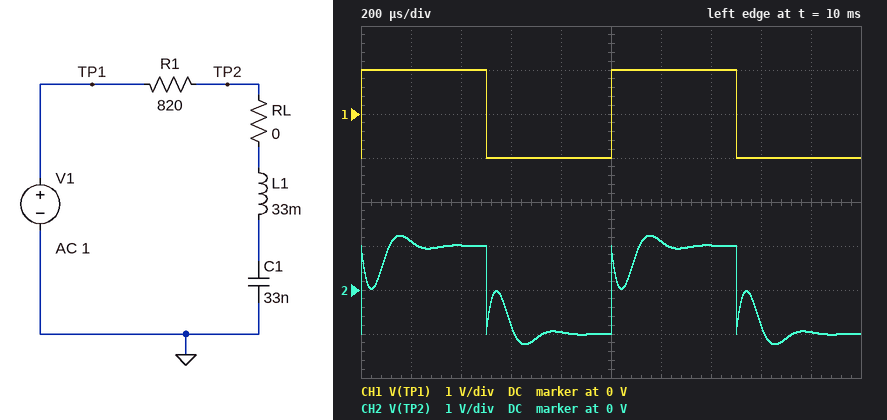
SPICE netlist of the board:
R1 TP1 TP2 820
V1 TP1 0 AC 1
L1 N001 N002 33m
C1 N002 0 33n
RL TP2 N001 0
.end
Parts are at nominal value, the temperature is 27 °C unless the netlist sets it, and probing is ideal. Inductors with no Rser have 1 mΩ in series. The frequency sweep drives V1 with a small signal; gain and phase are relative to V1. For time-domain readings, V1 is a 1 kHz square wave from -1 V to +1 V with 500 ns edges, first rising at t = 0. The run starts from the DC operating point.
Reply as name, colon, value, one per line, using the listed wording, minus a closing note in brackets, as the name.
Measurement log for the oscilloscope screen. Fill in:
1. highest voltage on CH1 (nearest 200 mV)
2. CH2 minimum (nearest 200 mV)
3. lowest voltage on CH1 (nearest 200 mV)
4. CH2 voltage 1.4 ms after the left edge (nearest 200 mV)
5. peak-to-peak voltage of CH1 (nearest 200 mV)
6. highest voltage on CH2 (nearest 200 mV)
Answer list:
highest voltage on CH1: 1.0 V
CH2 minimum: -1.2 V
lowest voltage on CH1: -1.0 V
CH2 voltage 1.4 ms after the left edge: 1.0 V
peak-to-peak voltage of CH1: 2.0 V
highest voltage on CH2: 1.2 V
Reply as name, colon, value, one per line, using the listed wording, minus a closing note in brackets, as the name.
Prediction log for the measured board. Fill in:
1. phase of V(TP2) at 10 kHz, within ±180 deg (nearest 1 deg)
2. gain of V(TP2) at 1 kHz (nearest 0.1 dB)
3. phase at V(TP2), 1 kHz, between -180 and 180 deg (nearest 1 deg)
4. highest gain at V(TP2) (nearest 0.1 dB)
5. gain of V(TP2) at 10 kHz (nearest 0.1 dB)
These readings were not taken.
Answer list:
phase of V(TP2) at 10 kHz, within ±180 deg: 27 deg
gain of V(TP2) at 1 kHz: -0.1 dB
phase at V(TP2), 1 kHz, between -180 and 180 deg: -10 deg
highest gain at V(TP2): 0 dB
gain of V(TP2) at 10 kHz: -1.0 dB
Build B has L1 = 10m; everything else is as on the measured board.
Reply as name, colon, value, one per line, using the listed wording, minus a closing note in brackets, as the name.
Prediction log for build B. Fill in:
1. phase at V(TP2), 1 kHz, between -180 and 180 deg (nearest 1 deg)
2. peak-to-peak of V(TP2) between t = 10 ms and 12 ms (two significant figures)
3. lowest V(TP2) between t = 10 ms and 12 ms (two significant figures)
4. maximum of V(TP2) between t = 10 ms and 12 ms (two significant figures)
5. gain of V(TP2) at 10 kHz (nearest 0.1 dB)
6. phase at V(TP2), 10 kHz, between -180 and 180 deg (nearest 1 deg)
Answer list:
phase at V(TP2), 1 kHz, between -180 and 180 deg: -10 deg
peak-to-peak of V(TP2) between t = 10 ms and 12 ms: 2.1 V
lowest V(TP2) between t = 10 ms and 12 ms: -1.0 V
maximum of V(TP2) between t = 10 ms and 12 ms: 1.0 V
gain of V(TP2) at 10 kHz: -15.1 dB
phase at V(TP2), 10 kHz, between -180 and 180 deg: 80 deg
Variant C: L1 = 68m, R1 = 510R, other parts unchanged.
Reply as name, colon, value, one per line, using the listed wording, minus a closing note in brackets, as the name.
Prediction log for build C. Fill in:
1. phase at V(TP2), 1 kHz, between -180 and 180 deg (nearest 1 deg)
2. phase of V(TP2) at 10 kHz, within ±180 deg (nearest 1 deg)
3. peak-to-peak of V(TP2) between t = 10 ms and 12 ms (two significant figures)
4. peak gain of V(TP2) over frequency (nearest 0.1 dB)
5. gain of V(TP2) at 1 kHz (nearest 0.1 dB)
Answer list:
phase at V(TP2), 1 kHz, between -180 and 180 deg: -7 deg
phase of V(TP2) at 10 kHz, within ±180 deg: 8 deg
peak-to-peak of V(TP2) between t = 10 ms and 12 ms: 2.7 V
peak gain of V(TP2) over frequency: 0 dB
gain of V(TP2) at 1 kHz: 0 dB
